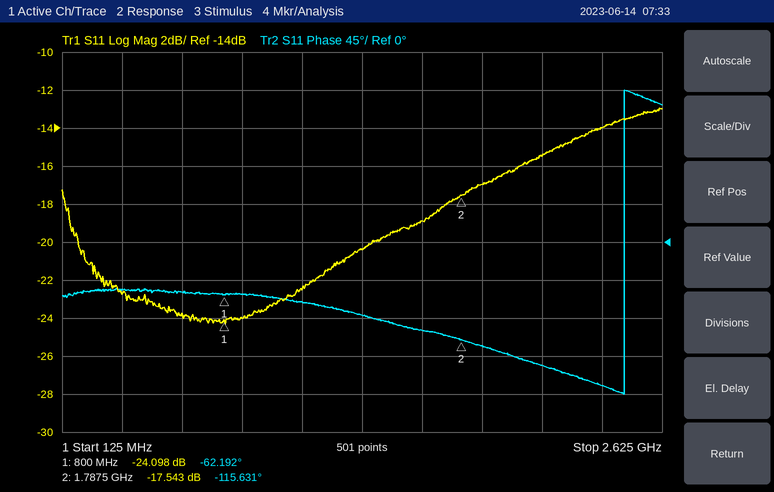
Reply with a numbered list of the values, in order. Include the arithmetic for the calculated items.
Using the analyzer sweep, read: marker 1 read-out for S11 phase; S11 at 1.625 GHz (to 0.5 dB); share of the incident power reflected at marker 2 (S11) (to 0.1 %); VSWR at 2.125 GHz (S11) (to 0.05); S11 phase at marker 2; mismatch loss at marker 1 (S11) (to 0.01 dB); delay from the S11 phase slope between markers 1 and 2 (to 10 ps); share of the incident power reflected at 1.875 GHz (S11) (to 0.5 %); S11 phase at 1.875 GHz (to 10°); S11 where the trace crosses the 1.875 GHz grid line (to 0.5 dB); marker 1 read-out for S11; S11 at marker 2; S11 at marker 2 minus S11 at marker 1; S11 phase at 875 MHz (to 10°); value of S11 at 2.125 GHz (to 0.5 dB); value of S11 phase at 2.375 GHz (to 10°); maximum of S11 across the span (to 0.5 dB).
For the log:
1. -62.192°
2. -19.0 dB
3. 10^(-17.543/10) ≈ 1.8 %
4. |Γ| = 10^(-15.5/20) = 0.1679; VSWR = (1 + 0.1679)/(1 − 0.1679) ≈ 1.40
5. -115.631°
6. −10 log10(1 − 10^(-24.098/10)) ≈ 0.02 dB
7. −(-115.631° − (-62.192°))/(360° × 987.5 MHz) ≈ 150 ps
8. 10^(-17/10) ≈ 2.0 %
9. -120°
10. -17.0 dB
11. -24.098 dB
12. -17.543 dB
13. -17.543 − (-24.098) = 6.555 dB
14. -60°
15. -15.5 dB
16. -170°
17. -13.0 dB
